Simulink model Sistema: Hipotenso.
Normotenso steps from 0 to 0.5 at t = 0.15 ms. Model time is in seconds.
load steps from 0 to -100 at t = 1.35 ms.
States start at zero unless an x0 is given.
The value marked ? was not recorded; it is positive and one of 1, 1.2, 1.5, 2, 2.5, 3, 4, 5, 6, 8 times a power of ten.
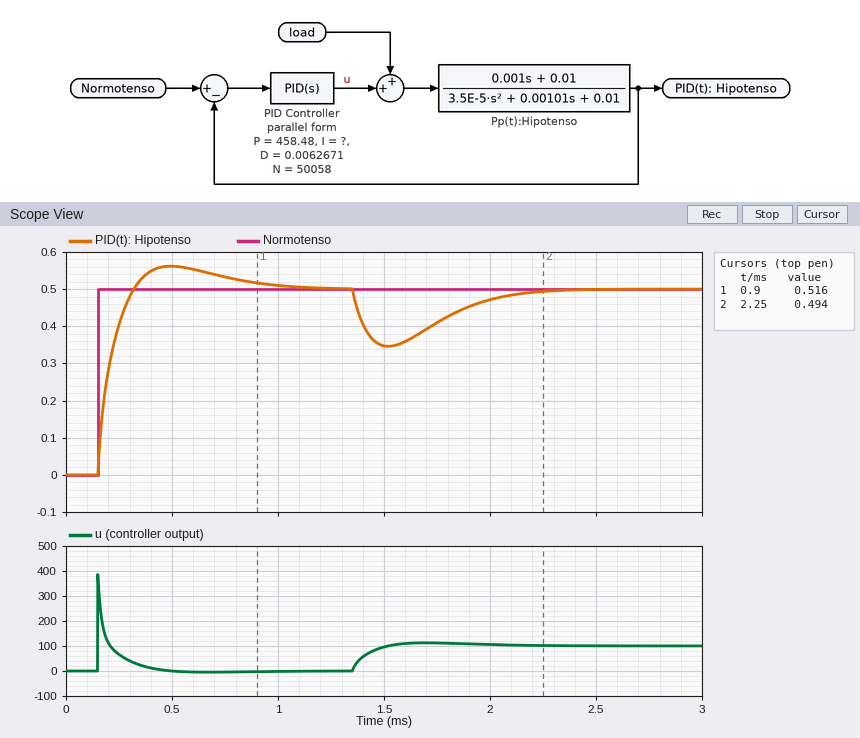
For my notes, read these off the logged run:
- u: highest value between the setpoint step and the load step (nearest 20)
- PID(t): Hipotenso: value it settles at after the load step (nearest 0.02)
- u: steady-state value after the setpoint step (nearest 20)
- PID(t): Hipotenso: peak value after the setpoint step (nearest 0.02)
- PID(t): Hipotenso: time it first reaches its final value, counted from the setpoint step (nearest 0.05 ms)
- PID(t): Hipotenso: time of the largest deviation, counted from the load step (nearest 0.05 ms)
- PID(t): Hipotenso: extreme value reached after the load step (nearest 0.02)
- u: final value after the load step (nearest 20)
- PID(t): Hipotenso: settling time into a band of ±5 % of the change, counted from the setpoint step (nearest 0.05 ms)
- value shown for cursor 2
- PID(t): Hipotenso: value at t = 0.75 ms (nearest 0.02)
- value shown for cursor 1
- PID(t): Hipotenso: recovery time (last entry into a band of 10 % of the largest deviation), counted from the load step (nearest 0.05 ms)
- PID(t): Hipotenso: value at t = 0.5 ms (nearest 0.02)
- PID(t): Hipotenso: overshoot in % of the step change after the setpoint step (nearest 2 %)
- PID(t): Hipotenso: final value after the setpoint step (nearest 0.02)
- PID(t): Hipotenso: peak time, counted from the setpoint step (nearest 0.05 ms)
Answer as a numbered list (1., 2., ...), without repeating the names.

1. 380
2. 0.50
3. 0
4. 0.56
5. 0.15 ms
6. 0.15 ms
7. 0.34
8. 100
9. 0.65 ms
10. 0.494
11. 0.54
12. 0.516
13. 0.75 ms
14. 0.56
15. 12 %
16. 0.50
17. 0.35 ms
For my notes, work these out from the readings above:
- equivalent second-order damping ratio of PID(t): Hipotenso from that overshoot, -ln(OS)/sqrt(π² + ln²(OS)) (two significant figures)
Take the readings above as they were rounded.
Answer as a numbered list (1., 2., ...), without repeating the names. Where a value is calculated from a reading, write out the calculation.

1. ln(0.12) = -2.120; 2.120 / sqrt(9.870 + 4.496) = 0.56
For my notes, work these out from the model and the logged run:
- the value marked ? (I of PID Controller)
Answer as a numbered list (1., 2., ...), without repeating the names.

1. 1.5e+06
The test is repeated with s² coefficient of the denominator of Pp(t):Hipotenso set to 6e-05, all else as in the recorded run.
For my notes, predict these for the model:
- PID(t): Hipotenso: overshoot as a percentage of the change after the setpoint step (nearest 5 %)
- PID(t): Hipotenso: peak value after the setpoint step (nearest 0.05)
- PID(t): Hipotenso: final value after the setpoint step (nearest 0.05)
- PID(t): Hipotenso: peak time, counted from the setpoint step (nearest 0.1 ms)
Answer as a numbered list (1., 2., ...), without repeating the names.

1. 20 %
2. 0.60
3. 0.50
4. 0.5 ms
